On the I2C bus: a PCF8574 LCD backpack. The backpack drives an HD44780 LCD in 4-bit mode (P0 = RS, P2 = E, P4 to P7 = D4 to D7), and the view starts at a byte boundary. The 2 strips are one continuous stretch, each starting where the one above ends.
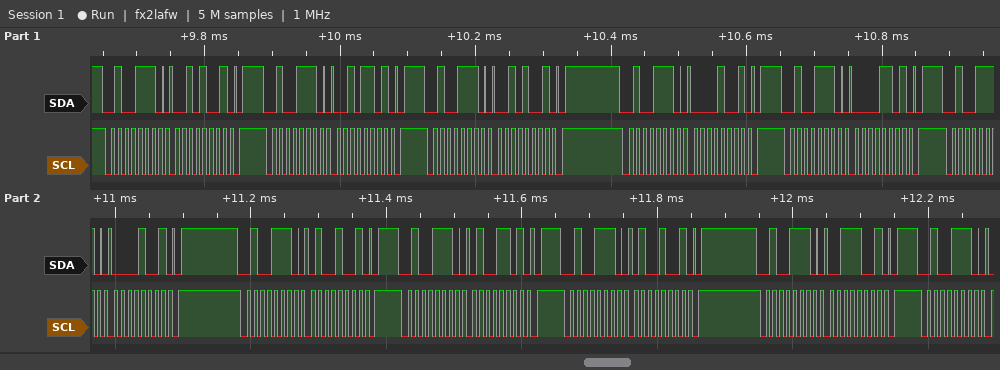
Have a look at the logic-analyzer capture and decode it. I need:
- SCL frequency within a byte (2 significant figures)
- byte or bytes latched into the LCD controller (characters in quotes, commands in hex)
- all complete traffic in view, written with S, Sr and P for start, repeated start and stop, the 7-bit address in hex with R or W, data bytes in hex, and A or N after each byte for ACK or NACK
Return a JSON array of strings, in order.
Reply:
["100 kHz", "' '", "S 27W A 29 A P S 27W A 2D A P S 27W A 29 A P S 27W A 09 A P S 27W A 0D A P S 27W A 09 A P S 27W A 49 A P S 27W A 4D A P S 27W A 49 A P S 27W A 39 A P S 27W A"]
